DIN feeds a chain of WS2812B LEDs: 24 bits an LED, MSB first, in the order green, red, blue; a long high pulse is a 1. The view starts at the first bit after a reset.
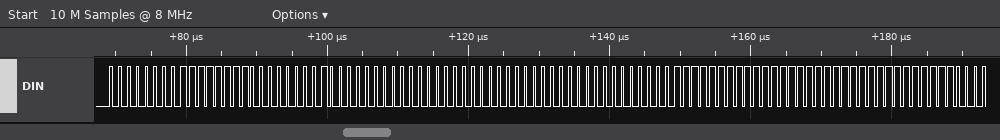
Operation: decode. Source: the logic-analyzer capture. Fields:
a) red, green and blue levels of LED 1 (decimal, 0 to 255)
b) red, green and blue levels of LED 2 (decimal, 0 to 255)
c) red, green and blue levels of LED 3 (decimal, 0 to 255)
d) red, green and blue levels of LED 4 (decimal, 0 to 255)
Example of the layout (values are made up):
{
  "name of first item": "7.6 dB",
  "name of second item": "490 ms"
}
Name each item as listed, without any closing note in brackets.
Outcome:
{
  "red, green and blue levels of LED 1": "255, 0, 0",
  "red, green and blue levels of LED 2": "0, 128, 0",
  "red, green and blue levels of LED 3": "0, 0, 255",
  "red, green and blue levels of LED 4": "255, 255, 255"
}
